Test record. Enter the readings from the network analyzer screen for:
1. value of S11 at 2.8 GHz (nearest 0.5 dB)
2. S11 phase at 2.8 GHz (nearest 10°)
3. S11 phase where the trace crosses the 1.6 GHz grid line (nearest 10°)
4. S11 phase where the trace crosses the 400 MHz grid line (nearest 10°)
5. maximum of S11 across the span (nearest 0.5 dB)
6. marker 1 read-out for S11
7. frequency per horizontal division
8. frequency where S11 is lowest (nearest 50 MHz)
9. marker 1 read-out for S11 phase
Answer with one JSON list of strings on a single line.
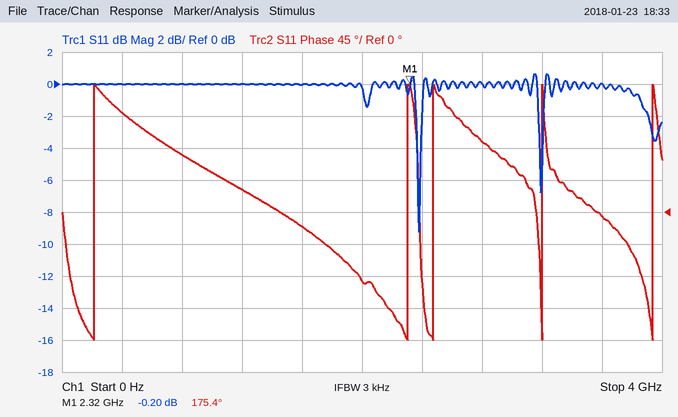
["0.0 dB", "100°", "-20°", "140°", "0.5 dB", "-0.20 dB", "400 MHz", "2.40 GHz", "175.4°"]
